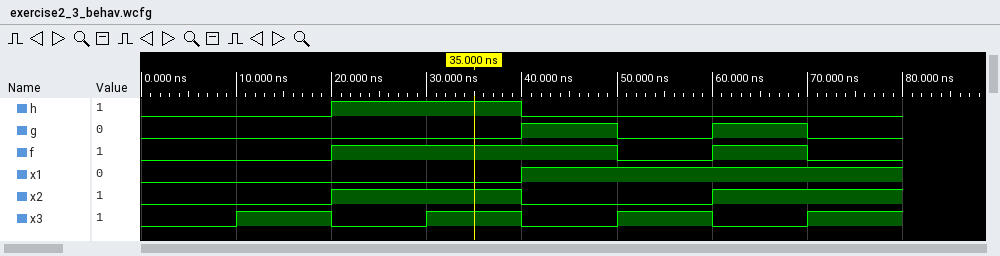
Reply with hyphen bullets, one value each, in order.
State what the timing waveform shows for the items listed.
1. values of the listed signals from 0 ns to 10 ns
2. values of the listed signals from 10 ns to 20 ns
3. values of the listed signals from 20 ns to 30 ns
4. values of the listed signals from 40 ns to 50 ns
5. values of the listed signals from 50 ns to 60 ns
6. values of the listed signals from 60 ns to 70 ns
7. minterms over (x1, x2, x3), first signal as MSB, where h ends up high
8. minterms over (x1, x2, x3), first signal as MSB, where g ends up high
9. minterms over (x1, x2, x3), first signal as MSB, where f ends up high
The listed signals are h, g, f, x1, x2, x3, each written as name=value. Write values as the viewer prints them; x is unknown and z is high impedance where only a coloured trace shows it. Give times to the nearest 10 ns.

- h=0, g=0, f=0, x1=0, x2=0, x3=0
- h=0, g=0, f=0, x1=0, x2=0, x3=1
- h=1, g=0, f=1, x1=0, x2=1, x3=0
- h=0, g=1, f=1, x1=1, x2=0, x3=0
- h=0, g=0, f=0, x1=1, x2=0, x3=1
- h=0, g=1, f=1, x1=1, x2=1, x3=0
- 2, 3
- 4, 6
- 2, 3, 4, 6
